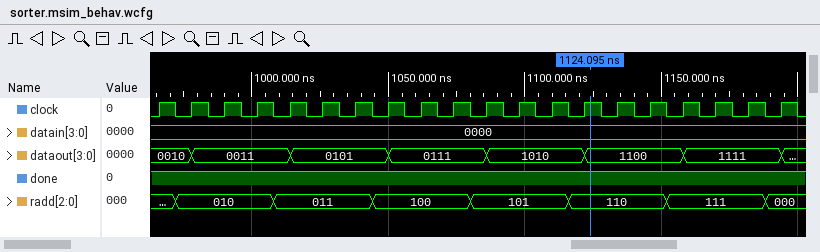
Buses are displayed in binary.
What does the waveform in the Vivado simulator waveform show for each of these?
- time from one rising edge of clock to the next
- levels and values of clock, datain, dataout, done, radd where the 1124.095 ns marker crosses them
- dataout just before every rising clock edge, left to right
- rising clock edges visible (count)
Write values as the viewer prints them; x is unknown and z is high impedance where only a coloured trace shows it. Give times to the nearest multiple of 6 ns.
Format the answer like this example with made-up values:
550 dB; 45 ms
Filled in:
12 ns; clock=1, datain=0000, dataout=1100, done=1, radd=110; 0010, 0010, 0011, 0011, 0011, 0101, 0101, 0101, 0111, 0111, 0111, 1010, 1010, 1010, 1100, 1100, 1100, 1111, 1111, 1111; 20
